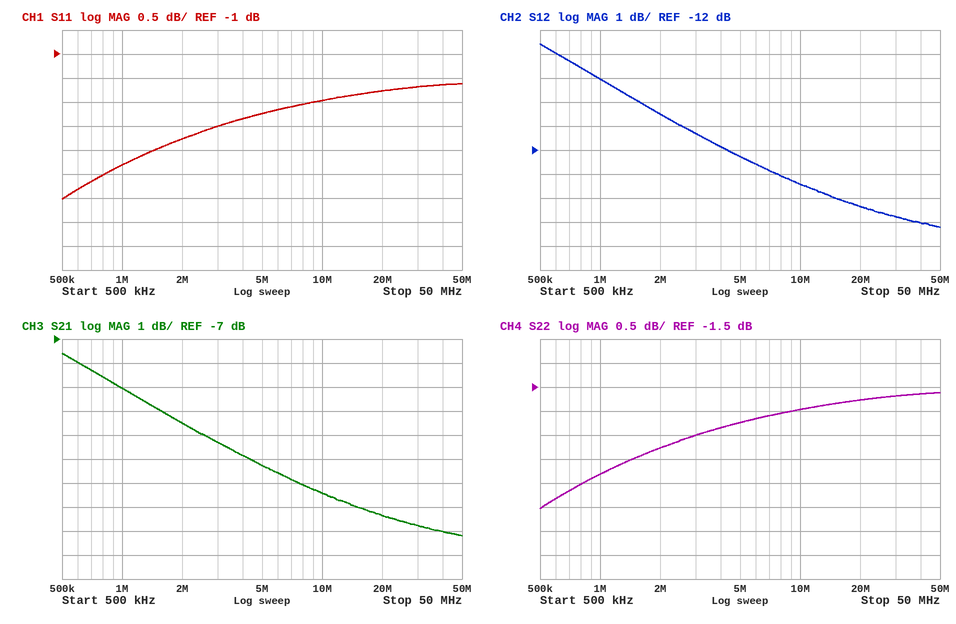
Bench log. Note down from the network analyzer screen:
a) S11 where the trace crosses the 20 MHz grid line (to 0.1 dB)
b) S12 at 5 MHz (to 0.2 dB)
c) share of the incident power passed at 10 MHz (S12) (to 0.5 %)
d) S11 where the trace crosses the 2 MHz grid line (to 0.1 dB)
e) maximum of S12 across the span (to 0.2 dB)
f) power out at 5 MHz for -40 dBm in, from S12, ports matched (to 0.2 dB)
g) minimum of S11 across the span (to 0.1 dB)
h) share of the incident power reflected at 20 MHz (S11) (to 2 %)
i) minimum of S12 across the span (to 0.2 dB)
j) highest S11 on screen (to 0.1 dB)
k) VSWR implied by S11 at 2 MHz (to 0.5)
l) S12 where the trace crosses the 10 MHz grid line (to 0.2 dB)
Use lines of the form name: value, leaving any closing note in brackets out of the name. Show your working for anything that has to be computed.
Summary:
S11 where the trace crosses the 20 MHz grid line: -1.8 dB
S12 at 5 MHz: -12.2 dB
share of the incident power passed at 10 MHz (S12): 10^(-13.4/10) ≈ 4.57 %, so 4.5 % to the nearest 0.5 %
S11 where the trace crosses the 2 MHz grid line: -2.8 dB
maximum of S12 across the span: -7.6 dB
power out at 5 MHz for -40 dBm in, from S12, ports matched: -40 dBm + (-12.2 dB) = -52.2 dBm
minimum of S11 across the span: -4.0 dB
share of the incident power reflected at 20 MHz (S11): 10^(-1.8/10) ≈ 66 %
minimum of S12 across the span: -15.2 dB
highest S11 on screen: -1.6 dB
VSWR implied by S11 at 2 MHz: |Γ| = 10^(-2.8/20) = 0.7244; VSWR = (1 + 0.7244)/(1 − 0.7244) ≈ 6.26, so 6.5 to the nearest 0.5
S12 where the trace crosses the 10 MHz grid line: -13.4 dB
